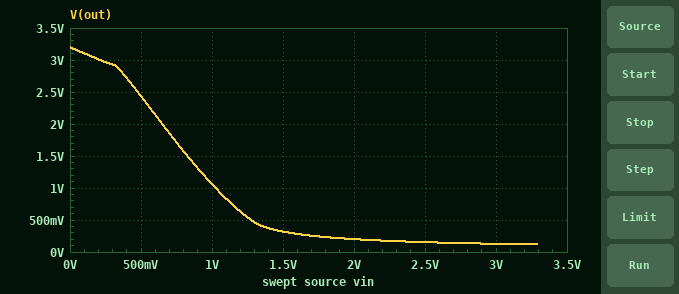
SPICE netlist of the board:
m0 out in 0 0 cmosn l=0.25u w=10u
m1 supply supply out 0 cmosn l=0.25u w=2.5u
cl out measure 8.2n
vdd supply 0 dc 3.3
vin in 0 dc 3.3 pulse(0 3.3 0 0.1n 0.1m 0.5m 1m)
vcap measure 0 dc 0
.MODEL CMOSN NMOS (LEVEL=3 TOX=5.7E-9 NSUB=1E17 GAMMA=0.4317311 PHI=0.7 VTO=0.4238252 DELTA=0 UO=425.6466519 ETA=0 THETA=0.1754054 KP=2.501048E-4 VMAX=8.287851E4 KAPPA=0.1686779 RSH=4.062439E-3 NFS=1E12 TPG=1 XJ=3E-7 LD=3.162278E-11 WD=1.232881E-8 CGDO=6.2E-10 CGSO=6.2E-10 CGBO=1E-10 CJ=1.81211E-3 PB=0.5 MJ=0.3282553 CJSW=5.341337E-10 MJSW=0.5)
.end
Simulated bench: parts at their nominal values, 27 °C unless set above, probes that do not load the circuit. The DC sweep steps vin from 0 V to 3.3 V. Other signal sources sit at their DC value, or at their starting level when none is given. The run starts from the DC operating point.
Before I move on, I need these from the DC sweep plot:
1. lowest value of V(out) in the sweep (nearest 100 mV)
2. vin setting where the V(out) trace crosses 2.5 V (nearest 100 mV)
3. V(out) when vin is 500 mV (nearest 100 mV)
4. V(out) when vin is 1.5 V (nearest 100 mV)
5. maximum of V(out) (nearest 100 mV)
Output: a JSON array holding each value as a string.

["100 mV", "500 mV", "2.4 V", "300 mV", "3.2 V"]
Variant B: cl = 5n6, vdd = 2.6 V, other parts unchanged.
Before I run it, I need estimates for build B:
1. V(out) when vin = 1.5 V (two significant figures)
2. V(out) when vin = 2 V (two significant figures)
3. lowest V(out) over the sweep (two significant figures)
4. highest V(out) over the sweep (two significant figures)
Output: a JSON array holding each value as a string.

["190 mV", "130 mV", "79 mV", "2.5 V"]
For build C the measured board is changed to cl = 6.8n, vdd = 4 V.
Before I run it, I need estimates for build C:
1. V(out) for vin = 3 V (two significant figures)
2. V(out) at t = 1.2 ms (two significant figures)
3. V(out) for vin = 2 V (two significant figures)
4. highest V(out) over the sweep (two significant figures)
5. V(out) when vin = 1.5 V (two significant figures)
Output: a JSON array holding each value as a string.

["180 mV", "160 mV", "300 mV", "3.9 V", "600 mV"]
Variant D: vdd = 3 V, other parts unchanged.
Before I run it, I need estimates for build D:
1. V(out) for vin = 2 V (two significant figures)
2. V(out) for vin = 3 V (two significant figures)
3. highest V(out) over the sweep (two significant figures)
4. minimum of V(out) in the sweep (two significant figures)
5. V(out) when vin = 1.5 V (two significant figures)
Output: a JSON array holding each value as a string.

["170 mV", "110 mV", "2.9 V", "100 mV", "250 mV"]
